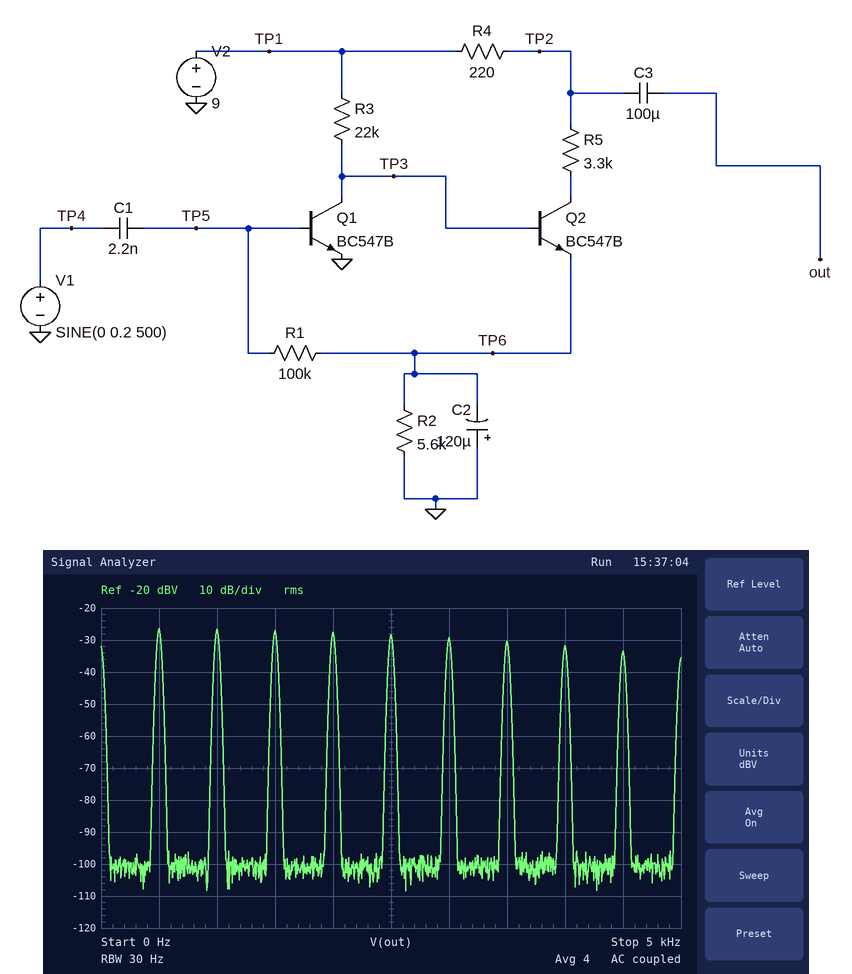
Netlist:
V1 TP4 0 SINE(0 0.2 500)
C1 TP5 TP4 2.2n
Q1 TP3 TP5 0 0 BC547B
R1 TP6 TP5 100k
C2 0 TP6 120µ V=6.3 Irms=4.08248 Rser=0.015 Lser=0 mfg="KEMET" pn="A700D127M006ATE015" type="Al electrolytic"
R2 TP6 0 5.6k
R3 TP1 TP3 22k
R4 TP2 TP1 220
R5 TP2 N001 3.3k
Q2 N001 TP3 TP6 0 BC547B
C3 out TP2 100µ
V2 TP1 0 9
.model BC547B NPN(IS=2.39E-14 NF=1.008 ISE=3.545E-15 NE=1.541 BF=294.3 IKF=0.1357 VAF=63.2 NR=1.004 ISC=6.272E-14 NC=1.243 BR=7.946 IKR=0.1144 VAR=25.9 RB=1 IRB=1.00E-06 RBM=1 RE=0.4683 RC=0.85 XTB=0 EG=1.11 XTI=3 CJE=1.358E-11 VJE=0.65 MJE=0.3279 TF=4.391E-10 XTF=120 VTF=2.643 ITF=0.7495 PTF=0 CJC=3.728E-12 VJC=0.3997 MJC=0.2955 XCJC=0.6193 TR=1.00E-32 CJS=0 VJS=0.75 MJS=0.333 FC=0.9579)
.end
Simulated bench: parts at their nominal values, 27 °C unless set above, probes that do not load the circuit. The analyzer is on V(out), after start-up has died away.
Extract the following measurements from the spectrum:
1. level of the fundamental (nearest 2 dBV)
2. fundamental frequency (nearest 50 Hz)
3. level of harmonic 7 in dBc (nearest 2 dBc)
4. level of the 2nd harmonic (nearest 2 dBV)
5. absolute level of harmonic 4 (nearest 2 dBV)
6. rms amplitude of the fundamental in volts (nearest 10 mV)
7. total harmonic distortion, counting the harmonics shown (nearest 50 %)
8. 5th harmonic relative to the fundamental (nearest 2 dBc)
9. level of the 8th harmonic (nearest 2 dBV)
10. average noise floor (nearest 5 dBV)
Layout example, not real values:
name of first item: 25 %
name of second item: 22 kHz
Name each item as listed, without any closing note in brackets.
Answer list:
level of the fundamental: -26 dBV
fundamental frequency: 500 Hz
level of harmonic 7 in dBc: -4 dBc
level of the 2nd harmonic: -26 dBV
absolute level of harmonic 4: -28 dBV
rms amplitude of the fundamental in volts: 50 mV
total harmonic distortion, counting the harmonics shown: 200 %
5th harmonic relative to the fundamental: -2 dBc
level of the 8th harmonic: -32 dBV
average noise floor: -100 dBV
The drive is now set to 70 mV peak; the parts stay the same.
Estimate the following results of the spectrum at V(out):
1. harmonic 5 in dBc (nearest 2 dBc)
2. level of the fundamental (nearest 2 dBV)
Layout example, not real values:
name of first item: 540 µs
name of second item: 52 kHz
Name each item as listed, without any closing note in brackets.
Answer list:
harmonic 5 in dBc: -4 dBc
level of the fundamental: -28 dBV
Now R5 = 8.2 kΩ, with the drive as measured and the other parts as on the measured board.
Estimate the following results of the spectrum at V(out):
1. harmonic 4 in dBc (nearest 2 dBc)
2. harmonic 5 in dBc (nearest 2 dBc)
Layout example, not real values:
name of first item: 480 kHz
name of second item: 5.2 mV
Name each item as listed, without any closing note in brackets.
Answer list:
harmonic 4 in dBc: -6 dBc
harmonic 5 in dBc: -12 dBc
